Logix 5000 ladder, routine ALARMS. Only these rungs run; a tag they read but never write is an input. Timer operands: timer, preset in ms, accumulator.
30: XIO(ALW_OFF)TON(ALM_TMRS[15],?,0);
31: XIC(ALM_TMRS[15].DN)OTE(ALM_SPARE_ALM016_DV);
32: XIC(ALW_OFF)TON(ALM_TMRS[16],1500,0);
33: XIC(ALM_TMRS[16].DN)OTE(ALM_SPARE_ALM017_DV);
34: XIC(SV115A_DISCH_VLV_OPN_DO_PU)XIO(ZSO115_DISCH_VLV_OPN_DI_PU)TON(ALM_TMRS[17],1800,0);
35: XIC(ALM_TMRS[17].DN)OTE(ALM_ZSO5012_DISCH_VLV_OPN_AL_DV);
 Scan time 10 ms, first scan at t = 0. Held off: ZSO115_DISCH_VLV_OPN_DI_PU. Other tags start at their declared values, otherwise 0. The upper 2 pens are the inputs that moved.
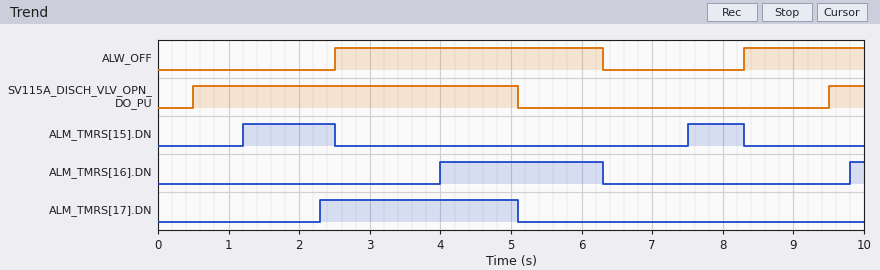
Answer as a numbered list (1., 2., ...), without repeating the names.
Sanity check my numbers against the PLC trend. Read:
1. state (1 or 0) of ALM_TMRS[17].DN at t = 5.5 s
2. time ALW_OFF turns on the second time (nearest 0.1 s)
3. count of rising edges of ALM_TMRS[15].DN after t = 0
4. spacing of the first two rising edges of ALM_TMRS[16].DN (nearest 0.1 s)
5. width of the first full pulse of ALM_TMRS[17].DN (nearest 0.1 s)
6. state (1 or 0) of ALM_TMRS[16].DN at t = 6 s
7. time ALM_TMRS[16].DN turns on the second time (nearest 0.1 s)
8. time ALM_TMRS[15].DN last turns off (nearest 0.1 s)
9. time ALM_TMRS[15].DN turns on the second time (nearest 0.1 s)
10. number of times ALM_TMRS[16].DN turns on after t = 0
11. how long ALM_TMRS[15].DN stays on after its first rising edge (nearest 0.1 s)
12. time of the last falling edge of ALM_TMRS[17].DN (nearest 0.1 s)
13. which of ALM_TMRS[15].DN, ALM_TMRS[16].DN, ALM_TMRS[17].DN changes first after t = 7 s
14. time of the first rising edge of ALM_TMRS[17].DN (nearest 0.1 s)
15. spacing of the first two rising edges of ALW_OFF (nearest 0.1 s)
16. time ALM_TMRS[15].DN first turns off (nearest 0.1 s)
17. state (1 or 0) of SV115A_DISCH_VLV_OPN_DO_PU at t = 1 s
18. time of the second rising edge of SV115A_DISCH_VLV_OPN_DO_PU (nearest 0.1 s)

1. 0
2. 8.3 s
3. 2
4. 5.8 s
5. 2.8 s
6. 1
7. 9.8 s
8. 8.3 s
9. 7.5 s
10. 2
11. 1.3 s
12. 5.1 s
13. ALM_TMRS[15].DN
14. 2.3 s
15. 5.8 s
16. 2.5 s
17. 1
18. 9.5 s
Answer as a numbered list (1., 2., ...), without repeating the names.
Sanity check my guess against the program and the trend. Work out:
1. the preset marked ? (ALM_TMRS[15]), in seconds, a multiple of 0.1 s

1. 1.2 s
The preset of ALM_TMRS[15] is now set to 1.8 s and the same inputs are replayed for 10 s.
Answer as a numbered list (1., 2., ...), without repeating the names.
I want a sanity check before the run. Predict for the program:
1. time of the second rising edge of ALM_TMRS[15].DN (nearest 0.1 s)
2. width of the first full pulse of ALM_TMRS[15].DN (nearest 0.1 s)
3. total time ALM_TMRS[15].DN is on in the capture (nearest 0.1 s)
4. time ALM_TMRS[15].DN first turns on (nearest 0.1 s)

1. 8.1 s
2. 0.7 s
3. 0.9 s
4. 1.8 s
